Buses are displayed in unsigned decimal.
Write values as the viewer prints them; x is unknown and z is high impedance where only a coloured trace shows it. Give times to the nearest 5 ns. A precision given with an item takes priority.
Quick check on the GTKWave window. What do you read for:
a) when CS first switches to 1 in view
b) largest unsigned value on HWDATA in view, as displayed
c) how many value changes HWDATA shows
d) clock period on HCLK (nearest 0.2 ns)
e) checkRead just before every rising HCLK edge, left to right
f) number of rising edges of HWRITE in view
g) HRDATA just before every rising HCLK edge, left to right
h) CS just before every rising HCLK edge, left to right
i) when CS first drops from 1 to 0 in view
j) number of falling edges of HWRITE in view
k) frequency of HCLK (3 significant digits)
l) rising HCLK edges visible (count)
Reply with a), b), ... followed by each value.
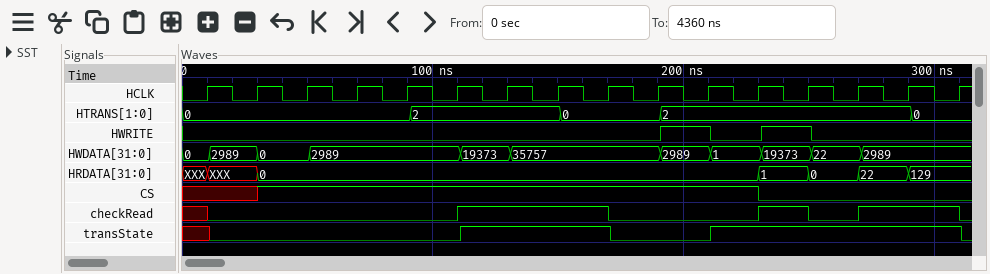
a) 30 ns
b) 35757
c) 10
d) 20 ns
e) x 0 0 0 0 0 1 1 1 0 0 0 1 0 1 1
f) 2
g) XXX, XXX, 0, 0, 0, 0, 0, 0, 0, 0, 0, 0, 1, 0, 22, 129
h) x x 1 1 1 1 1 1 1 1 1 1 0 0 0 0
i) 230 ns
j) 2
k) 50.0 MHz
l) 16
